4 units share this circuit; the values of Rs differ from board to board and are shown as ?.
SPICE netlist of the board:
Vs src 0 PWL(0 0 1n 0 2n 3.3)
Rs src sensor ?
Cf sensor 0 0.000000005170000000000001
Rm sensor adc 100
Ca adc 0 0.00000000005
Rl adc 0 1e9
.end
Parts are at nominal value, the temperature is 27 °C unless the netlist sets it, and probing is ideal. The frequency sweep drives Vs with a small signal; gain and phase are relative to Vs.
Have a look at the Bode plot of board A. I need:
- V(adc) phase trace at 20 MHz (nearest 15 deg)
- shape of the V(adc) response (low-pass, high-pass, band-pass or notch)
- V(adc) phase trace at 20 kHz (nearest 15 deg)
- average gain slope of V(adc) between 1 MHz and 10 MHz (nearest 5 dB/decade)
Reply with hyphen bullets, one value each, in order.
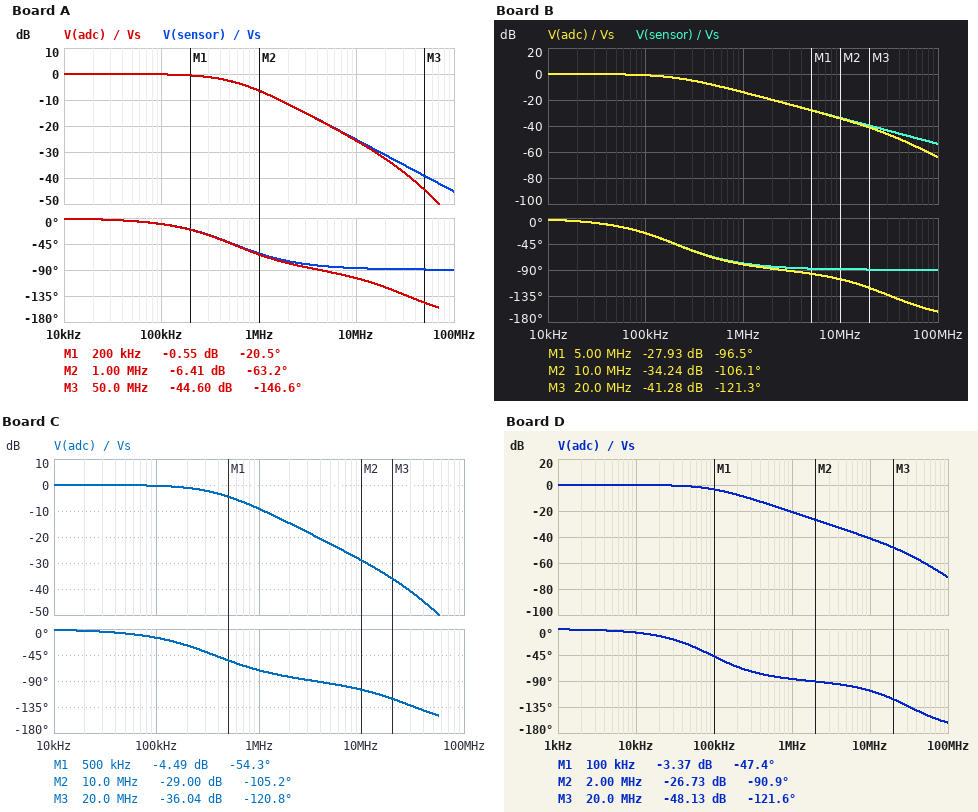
- -120 deg
- low-pass
- 0 deg
- -20 dB/decade
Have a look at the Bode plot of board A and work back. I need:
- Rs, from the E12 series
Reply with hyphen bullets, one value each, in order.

- 56 Ω
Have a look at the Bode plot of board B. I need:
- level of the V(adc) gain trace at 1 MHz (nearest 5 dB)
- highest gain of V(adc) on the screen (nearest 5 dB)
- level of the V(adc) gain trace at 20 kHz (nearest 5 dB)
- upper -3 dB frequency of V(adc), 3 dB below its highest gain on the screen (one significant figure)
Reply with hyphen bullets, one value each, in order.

- -15 dB
- 0 dB
- 0 dB
- 200 kHz
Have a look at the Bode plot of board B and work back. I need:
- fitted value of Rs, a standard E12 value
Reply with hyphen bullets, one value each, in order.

- 150 Ω
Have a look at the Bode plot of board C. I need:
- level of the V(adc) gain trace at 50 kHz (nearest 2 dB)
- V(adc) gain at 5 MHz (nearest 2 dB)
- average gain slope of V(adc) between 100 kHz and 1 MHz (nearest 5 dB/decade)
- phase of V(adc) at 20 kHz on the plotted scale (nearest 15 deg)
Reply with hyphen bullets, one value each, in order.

- 0 dB
- -22 dB
- -10 dB/decade
- 0 deg
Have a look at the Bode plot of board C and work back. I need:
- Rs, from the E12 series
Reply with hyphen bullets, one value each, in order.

- 82 Ω
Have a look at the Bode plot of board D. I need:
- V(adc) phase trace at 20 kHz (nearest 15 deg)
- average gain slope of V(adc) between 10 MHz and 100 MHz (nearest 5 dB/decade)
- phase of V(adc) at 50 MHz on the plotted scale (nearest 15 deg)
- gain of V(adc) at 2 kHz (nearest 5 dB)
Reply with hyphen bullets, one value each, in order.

- -15 deg
- -30 dB/decade
- -150 deg
- 0 dB
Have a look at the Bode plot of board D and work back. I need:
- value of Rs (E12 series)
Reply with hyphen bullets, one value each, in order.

- 330 Ω
